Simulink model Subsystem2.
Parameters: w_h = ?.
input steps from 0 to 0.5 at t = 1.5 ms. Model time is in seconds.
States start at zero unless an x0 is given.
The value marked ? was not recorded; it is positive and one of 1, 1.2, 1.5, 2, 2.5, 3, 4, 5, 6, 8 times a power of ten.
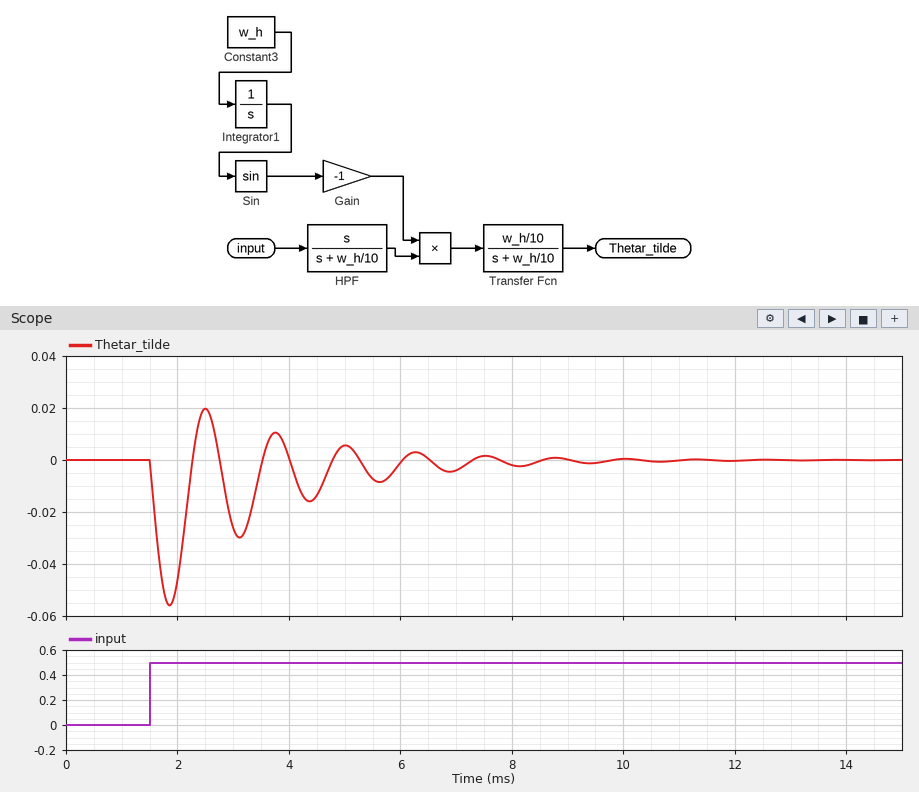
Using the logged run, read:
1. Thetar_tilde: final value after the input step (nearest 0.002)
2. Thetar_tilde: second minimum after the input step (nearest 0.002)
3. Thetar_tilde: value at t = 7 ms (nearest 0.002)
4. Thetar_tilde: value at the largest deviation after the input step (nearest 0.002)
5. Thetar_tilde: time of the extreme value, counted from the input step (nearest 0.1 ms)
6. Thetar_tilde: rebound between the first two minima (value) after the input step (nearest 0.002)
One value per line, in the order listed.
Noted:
0.000
-0.030
-0.004
-0.056
0.4 ms
0.020
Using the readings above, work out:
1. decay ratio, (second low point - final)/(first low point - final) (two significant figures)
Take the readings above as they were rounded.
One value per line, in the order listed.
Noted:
0.54
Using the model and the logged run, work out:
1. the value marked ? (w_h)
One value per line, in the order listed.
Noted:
5000
